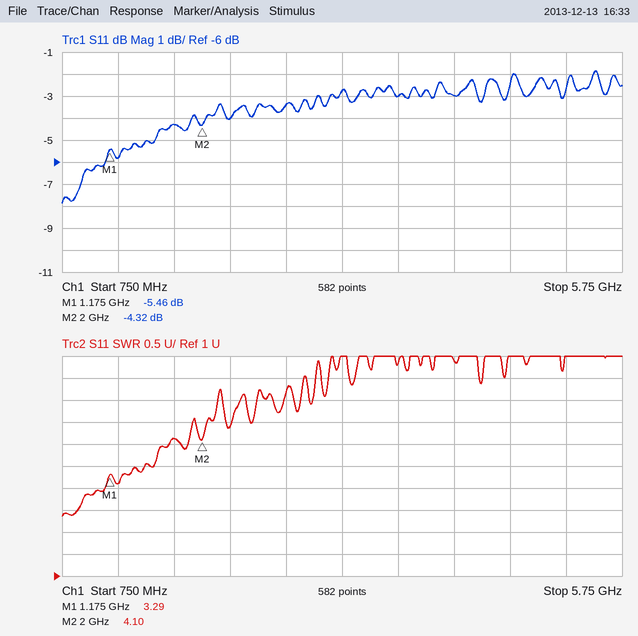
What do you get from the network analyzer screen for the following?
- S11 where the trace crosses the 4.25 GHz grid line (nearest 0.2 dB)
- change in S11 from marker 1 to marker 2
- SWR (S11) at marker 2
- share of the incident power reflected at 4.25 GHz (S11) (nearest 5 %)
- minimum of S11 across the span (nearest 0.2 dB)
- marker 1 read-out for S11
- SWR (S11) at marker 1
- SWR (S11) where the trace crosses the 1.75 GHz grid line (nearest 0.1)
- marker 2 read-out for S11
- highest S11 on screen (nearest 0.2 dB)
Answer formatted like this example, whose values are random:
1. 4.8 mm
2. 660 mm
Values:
1. -3.0 dB
2. 1.14 dB
3. 4.10
4. 50 %
5. -7.8 dB
6. -5.46 dB
7. 3.29
8. 4.1
9. -4.32 dB
10. -1.8 dB
